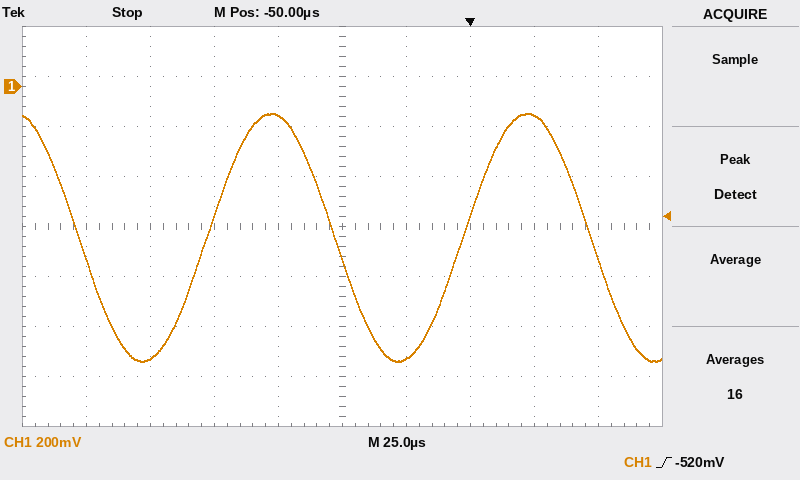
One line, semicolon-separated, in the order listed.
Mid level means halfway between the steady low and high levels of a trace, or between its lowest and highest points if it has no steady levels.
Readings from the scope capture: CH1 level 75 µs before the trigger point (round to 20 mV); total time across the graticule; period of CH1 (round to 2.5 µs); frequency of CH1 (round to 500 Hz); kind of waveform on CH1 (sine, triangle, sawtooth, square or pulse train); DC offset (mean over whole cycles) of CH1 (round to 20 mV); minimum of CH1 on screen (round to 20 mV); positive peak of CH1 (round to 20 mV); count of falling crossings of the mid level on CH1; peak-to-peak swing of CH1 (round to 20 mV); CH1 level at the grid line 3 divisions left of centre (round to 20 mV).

-120 mV; 250 µs; 100.0 µs; 10.0 kHz; sine; -600 mV; -1.10 V; -100 mV; 3; 1.00 V; -1.08 V
